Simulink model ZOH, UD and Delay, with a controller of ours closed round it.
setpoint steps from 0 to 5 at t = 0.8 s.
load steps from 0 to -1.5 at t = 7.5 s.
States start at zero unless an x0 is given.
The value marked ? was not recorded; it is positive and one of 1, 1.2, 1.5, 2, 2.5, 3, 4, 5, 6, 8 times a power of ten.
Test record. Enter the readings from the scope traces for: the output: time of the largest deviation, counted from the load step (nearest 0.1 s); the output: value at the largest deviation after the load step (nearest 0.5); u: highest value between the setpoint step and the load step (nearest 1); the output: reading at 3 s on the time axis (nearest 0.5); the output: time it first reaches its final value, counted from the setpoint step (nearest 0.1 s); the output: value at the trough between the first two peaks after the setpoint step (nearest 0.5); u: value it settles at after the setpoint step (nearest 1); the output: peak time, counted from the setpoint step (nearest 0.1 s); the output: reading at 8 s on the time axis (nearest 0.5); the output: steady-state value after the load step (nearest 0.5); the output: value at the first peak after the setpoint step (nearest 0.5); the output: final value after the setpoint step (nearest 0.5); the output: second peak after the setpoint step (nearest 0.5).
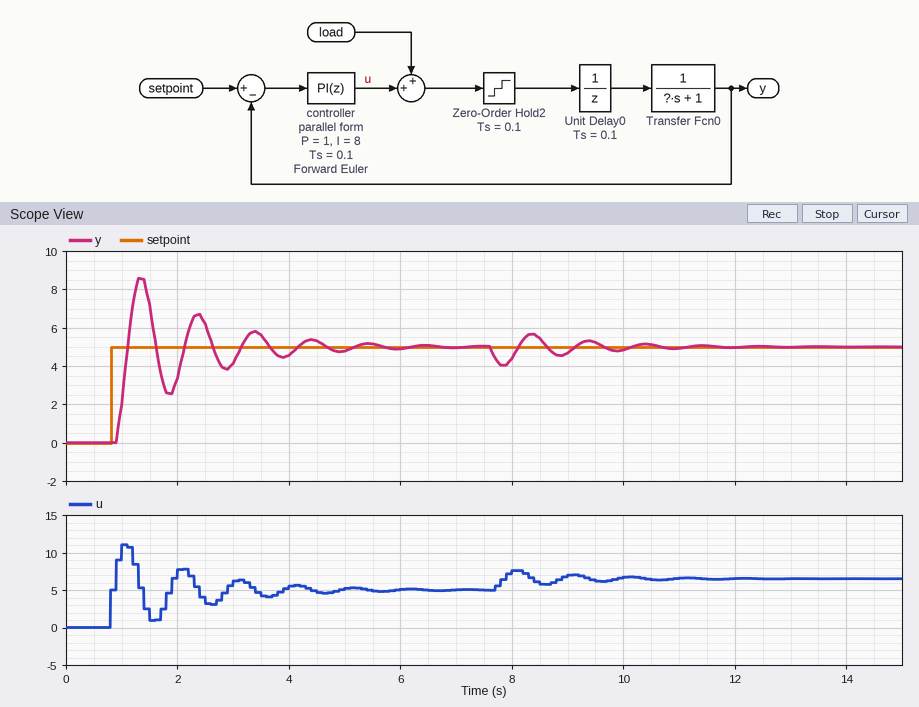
0.3 s
4.0
11
4.0
0.3 s
2.5
5
0.5 s
4.5
5.0
8.5
5.0
6.5
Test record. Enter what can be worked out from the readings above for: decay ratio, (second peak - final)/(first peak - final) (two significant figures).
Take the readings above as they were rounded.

0.43
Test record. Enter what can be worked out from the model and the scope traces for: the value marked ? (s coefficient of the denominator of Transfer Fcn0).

0.2
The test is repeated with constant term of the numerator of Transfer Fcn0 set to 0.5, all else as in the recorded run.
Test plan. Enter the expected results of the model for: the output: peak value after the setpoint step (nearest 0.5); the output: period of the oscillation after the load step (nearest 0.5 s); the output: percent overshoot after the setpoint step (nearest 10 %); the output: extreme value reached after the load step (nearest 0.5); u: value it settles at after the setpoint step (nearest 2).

6.5
1.5 s
30 %
4.5
10
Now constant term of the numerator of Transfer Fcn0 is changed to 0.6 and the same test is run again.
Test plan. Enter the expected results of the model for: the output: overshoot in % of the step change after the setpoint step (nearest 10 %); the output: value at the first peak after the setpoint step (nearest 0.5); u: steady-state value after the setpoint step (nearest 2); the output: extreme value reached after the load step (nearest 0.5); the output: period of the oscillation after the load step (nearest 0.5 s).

40 %
7.0
8
4.5
1.5 s
